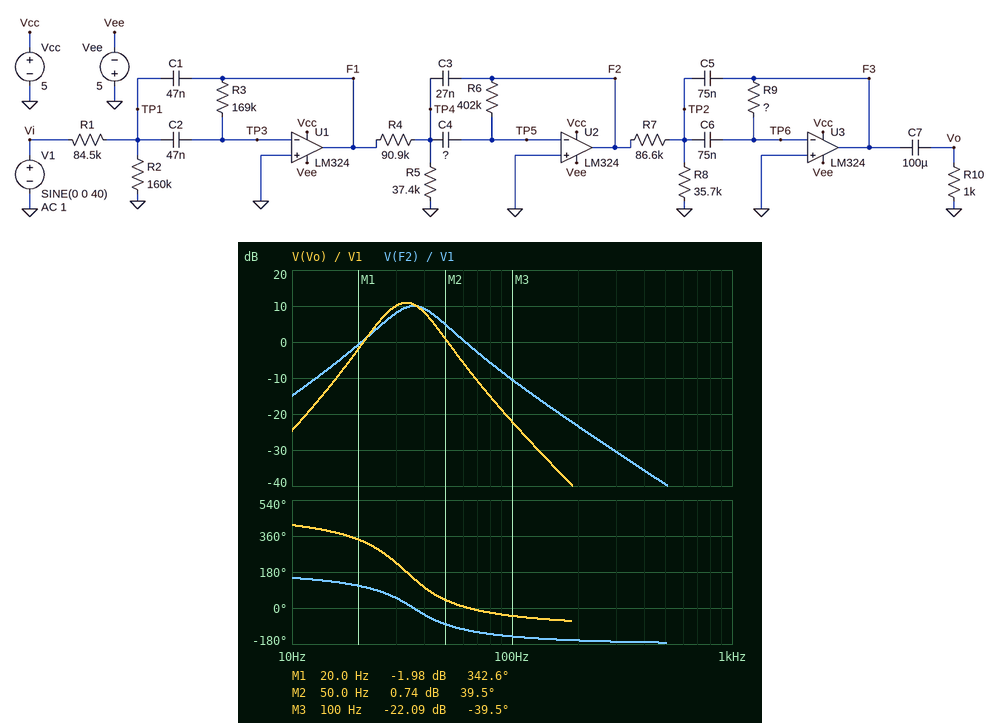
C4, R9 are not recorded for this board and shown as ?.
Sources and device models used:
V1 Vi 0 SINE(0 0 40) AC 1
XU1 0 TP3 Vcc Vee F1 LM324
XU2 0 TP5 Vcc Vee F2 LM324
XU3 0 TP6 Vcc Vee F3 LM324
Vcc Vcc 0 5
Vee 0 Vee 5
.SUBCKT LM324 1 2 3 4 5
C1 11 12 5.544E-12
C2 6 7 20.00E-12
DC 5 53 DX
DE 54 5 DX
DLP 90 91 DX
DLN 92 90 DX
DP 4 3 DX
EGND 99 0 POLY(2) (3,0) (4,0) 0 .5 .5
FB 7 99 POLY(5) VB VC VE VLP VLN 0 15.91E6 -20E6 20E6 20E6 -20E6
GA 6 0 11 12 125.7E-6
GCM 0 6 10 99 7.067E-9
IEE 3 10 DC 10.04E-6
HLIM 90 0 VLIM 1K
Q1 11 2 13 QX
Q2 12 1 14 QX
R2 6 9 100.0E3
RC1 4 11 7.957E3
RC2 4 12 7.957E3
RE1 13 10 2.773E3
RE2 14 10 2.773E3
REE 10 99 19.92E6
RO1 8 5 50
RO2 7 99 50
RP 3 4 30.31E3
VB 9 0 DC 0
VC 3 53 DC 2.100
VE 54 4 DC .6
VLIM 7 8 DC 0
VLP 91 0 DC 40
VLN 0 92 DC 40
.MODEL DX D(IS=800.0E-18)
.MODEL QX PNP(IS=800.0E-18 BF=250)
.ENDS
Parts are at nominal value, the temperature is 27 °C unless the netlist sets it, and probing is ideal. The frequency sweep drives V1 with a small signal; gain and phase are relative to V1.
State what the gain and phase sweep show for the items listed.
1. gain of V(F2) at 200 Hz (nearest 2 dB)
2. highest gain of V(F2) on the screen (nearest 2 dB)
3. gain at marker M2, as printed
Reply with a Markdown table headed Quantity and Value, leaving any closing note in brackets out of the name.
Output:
| Quantity | Value |
|---|---|
| gain of V(F2) at 200 Hz | -24 dB |
| highest gain of V(F2) on the screen | 10 dB |
| gain at marker M2, as printed | 0.74 dB |
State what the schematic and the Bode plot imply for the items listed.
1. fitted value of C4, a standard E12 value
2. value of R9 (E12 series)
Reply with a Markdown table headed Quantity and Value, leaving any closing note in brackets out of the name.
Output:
| Quantity | Value |
|---|---|
| fitted value of C4, a standard E12 value | 68 nF |
| value of R9 | 220 kΩ |
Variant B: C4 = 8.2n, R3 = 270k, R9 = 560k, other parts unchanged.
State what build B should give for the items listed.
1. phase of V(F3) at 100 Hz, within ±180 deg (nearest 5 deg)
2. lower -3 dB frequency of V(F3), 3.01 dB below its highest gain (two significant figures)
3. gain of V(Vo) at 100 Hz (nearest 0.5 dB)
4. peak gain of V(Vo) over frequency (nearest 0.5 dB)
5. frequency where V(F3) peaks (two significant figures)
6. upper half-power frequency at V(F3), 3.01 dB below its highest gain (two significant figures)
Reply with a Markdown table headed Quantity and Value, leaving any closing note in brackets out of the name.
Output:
| Quantity | Value |
|---|---|
| phase of V(F3) at 100 Hz, within ±180 deg | 25 deg |
| lower -3 dB frequency of V(F3), 3.01 dB below its highest gain | 17 Hz |
| gain of V(Vo) at 100 Hz | -19.5 dB |
| peak gain of V(Vo) over frequency | -7.0 dB |
| frequency where V(F3) peaks | 20 Hz |
| upper half-power frequency at V(F3), 3.01 dB below its highest gain | 33 Hz |
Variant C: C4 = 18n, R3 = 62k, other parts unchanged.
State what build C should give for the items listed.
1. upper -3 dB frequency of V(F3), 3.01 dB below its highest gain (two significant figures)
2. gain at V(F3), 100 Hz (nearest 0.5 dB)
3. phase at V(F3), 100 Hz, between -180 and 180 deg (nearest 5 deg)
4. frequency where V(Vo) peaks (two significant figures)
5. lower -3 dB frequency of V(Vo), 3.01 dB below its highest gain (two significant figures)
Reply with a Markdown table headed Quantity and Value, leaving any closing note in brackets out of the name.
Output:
| Quantity | Value |
|---|---|
| upper -3 dB frequency of V(F3), 3.01 dB below its highest gain | 79 Hz |
| gain at V(F3), 100 Hz | -21.5 dB |
| phase at V(F3), 100 Hz, between -180 and 180 deg | 15 deg |
| frequency where V(Vo) peaks | 62 Hz |
| lower -3 dB frequency of V(Vo), 3.01 dB below its highest gain | 33 Hz |
